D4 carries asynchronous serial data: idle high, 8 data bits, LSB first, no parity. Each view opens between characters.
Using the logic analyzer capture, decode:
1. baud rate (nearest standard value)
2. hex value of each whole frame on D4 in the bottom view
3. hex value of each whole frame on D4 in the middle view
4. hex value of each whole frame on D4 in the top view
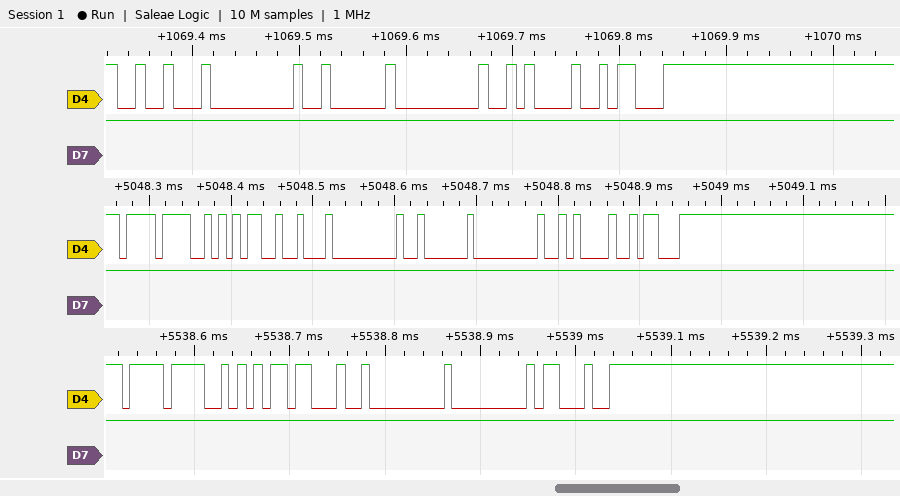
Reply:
115200 baud
EF, AA, 23, 00, 00, 23
EF, AA, 12, 00, 02, 00, 0A, 1A
12, 00, 02, 00, 0A, 1A
